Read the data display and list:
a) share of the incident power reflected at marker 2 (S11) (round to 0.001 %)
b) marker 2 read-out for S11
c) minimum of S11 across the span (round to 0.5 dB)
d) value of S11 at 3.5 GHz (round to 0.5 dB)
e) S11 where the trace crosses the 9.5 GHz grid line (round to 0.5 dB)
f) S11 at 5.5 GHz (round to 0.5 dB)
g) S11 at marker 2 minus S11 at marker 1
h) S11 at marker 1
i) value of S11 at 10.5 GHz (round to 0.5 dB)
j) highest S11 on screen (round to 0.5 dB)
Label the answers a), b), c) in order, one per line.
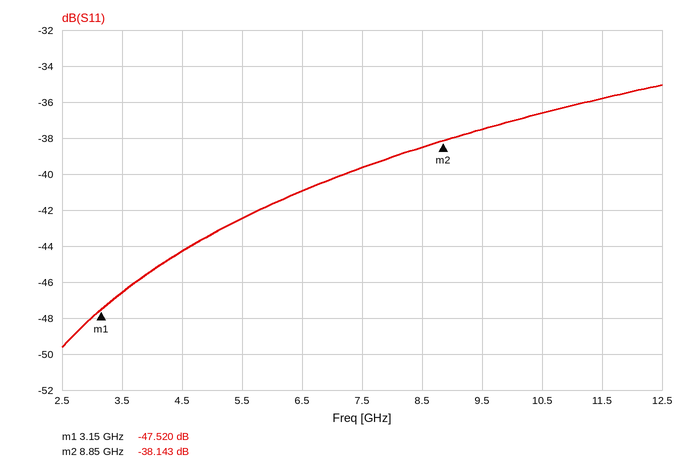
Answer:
a) 0.015 %
b) -38.143 dB
c) -49.5 dB
d) -46.5 dB
e) -37.5 dB
f) -42.5 dB
g) 9.377 dB
h) -47.520 dB
i) -36.5 dB
j) -35.0 dB
